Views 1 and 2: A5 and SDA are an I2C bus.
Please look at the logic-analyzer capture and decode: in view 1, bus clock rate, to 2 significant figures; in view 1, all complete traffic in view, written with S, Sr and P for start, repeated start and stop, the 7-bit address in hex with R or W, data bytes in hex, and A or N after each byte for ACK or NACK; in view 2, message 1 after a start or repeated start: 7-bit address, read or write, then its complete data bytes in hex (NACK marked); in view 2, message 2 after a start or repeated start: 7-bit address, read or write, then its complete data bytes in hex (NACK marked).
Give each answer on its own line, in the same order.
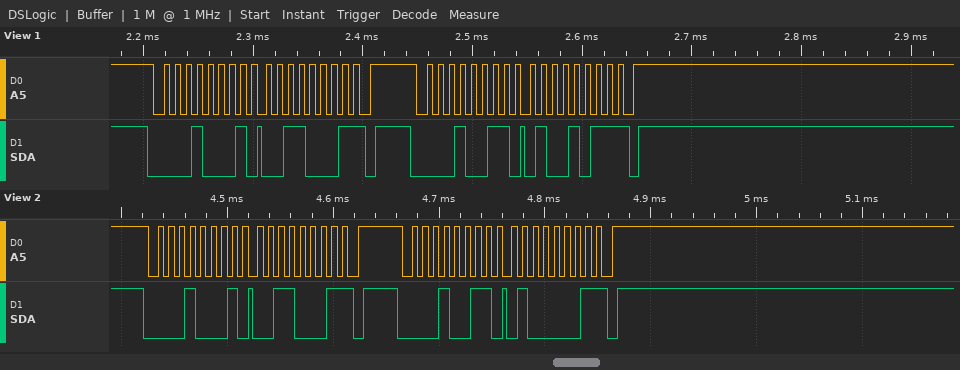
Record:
100 kHz
S 08R A 31 N P S 09R A 4B N P
0x08 read: 31 NACK
0x09 read: 41 NACK
